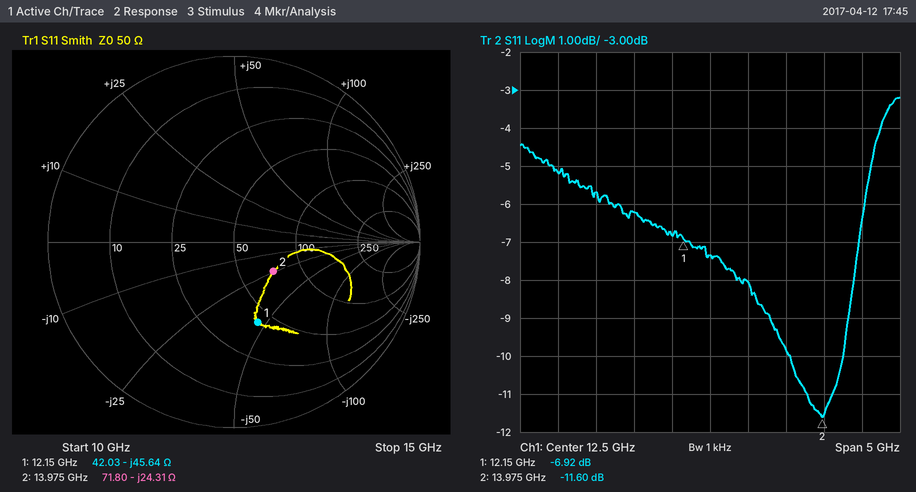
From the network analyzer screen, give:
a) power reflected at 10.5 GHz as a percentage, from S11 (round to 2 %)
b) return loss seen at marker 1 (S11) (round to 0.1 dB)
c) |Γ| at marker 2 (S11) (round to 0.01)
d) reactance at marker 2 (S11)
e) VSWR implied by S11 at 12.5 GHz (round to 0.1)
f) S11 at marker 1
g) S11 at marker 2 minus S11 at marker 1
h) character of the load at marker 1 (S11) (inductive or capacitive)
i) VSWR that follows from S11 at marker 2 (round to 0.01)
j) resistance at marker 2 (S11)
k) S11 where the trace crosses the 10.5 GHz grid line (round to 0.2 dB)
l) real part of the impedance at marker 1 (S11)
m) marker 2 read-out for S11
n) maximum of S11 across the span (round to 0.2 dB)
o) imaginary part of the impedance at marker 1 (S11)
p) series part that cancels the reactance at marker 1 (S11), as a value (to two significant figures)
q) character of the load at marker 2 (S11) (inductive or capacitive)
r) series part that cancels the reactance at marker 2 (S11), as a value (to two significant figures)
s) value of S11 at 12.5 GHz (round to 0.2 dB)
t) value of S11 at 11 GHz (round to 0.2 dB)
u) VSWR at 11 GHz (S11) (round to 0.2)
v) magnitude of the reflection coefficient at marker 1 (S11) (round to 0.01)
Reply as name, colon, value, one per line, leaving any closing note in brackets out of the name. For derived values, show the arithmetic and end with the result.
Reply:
power reflected at 10.5 GHz as a percentage, from S11: 10^(-5.2/10) ≈ 30 %
return loss seen at marker 1 (S11): 6.9 dB
|Γ| at marker 2 (S11): 0.26
reactance at marker 2: -24.31 Ω
VSWR implied by S11 at 12.5 GHz: |Γ| = 10^(-7.4/20) = 0.4266; VSWR = (1 + 0.4266)/(1 − 0.4266) ≈ 2.5
S11 at marker 1: -6.92 dB
S11 at marker 2 minus S11 at marker 1: -11.6 − (-6.92) = -4.68 dB
character of the load at marker 1 (S11): capacitive
VSWR that follows from S11 at marker 2: (1 + 0.2630)/(1 − 0.2630) ≈ 1.71
resistance at marker 2: 71.80 Ω
S11 where the trace crosses the 10.5 GHz grid line: -5.2 dB
real part of the impedance at marker 1: 42.03 Ω
marker 2 read-out for S11: -11.60 dB
maximum of S11 across the span: -3.2 dB
imaginary part of the impedance at marker 1: -45.64 Ω
series part that cancels the reactance at marker 1 (S11), as a value: L = 45.64 Ω/(2π × 12.15 GHz) ≈ 598 pH, so 600 pH to two significant figures
character of the load at marker 2 (S11): capacitive
series part that cancels the reactance at marker 2 (S11), as a value: L = 24.31 Ω/(2π × 13.975 GHz) ≈ 277 pH, so 280 pH to two significant figures
value of S11 at 12.5 GHz: -7.4 dB
value of S11 at 11 GHz: -5.6 dB
VSWR at 11 GHz (S11): |Γ| = 10^(-5.6/20) = 0.5248; VSWR = (1 + 0.5248)/(1 − 0.5248) ≈ 3.2
magnitude of the reflection coefficient at marker 1 (S11): 10^(-6.92/20) ≈ 0.45
